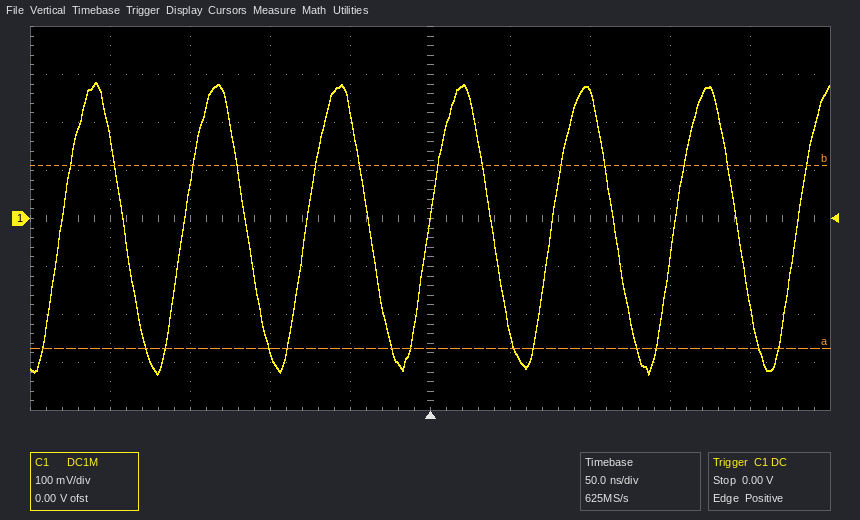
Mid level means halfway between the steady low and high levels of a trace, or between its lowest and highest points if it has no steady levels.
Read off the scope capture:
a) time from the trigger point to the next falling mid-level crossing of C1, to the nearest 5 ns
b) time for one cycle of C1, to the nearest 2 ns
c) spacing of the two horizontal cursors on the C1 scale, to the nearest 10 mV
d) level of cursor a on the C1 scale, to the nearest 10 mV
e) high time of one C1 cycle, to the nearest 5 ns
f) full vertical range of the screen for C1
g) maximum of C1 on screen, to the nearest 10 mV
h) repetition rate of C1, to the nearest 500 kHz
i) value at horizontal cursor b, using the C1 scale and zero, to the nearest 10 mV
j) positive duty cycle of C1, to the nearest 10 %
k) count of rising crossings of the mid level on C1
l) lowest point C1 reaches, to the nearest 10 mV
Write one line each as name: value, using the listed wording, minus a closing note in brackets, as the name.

time from the trigger point to the next falling mid-level crossing of C1, to the nearest 5 ns: 40 ns
time for one cycle of C1, to the nearest 2 ns: 76 ns
spacing of the two horizontal cursors on the C1 scale, to the nearest 10 mV: 380 mV
level of cursor a on the C1 scale, to the nearest 10 mV: -270 mV
high time of one C1 cycle, to the nearest 5 ns: 40 ns
full vertical range of the screen for C1: 800 mV
maximum of C1 on screen, to the nearest 10 mV: 280 mV
repetition rate of C1, to the nearest 500 kHz: 13.0 MHz
value at horizontal cursor b, using the C1 scale and zero, to the nearest 10 mV: 110 mV
positive duty cycle of C1, to the nearest 10 %: 50 %
count of rising crossings of the mid level on C1: 7
lowest point C1 reaches, to the nearest 10 mV: -320 mV
